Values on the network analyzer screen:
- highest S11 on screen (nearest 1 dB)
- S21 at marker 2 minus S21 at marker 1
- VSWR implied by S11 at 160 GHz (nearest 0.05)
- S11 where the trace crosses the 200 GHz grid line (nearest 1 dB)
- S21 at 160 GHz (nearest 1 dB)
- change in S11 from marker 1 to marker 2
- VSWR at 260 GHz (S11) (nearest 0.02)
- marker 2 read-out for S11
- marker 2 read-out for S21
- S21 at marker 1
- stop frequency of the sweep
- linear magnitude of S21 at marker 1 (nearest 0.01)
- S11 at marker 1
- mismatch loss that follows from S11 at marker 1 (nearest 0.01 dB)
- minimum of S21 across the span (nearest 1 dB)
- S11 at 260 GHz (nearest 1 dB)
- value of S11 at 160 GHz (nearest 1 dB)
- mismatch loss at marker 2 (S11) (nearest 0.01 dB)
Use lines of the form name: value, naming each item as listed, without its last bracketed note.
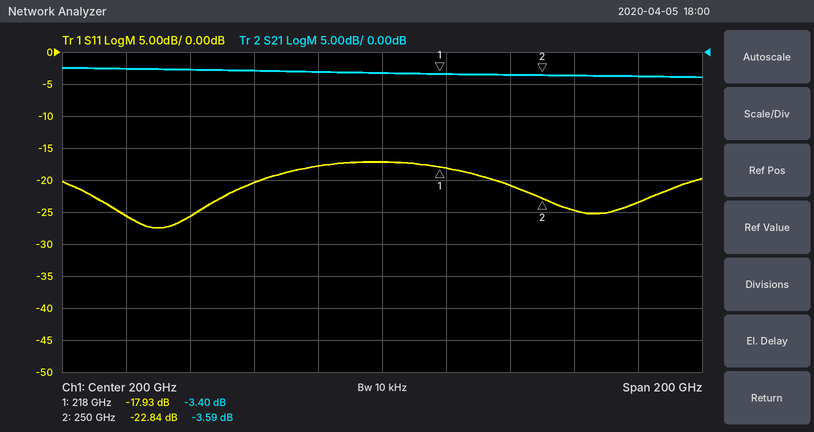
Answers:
highest S11 on screen: -17 dB
S21 at marker 2 minus S21 at marker 1: -0.19 dB
VSWR implied by S11 at 160 GHz: 1.20
S11 where the trace crosses the 200 GHz grid line: -17 dB
S21 at 160 GHz: -3 dB
change in S11 from marker 1 to marker 2: -4.91 dB
VSWR at 260 GHz (S11): 1.12
marker 2 read-out for S11: -22.84 dB
marker 2 read-out for S21: -3.59 dB
S21 at marker 1: -3.40 dB
stop frequency of the sweep: 300 GHz
linear magnitude of S21 at marker 1: 0.68
S11 at marker 1: -17.93 dB
mismatch loss that follows from S11 at marker 1: 0.07 dB
minimum of S21 across the span: -4 dB
S11 at 260 GHz: -25 dB
value of S11 at 160 GHz: -20 dB
mismatch loss at marker 2 (S11): 0.02 dB
